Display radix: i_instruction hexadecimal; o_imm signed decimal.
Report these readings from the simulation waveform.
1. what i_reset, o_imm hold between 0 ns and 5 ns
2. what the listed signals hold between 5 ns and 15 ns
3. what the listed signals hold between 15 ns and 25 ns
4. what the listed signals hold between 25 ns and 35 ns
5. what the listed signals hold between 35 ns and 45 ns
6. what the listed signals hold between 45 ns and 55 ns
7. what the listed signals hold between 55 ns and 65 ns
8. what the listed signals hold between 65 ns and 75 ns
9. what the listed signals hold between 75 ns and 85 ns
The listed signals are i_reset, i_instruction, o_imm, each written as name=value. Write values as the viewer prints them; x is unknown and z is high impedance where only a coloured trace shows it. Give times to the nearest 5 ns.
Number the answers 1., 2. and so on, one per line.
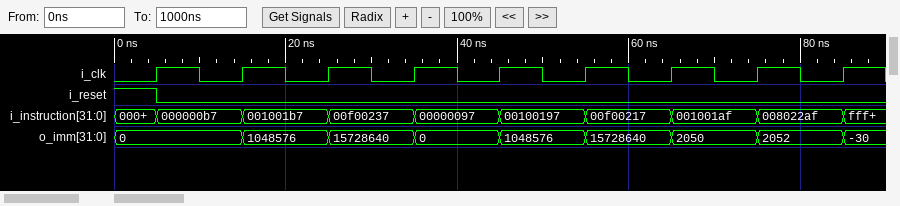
1. i_reset=1, o_imm=0
2. i_reset=0, i_instruction=000000b7, o_imm=0
3. i_reset=0, i_instruction=001001b7, o_imm=1048576
4. i_reset=0, i_instruction=00f00237, o_imm=15728640
5. i_reset=0, i_instruction=00000097, o_imm=0
6. i_reset=0, i_instruction=00100197, o_imm=1048576
7. i_reset=0, i_instruction=00f00217, o_imm=15728640
8. i_reset=0, i_instruction=001001af, o_imm=2050
9. i_reset=0, i_instruction=008022af, o_imm=2052
